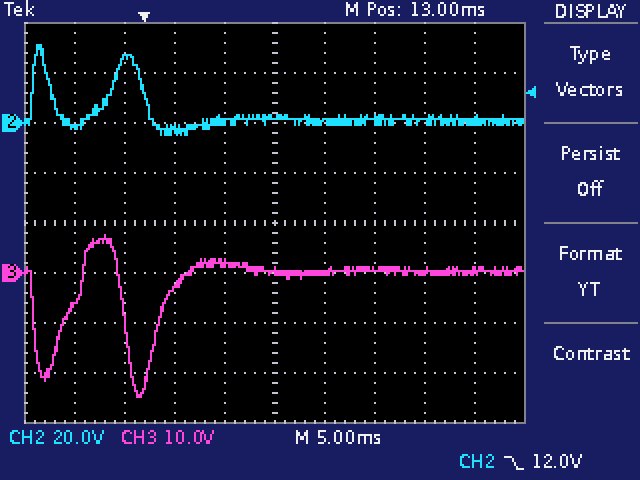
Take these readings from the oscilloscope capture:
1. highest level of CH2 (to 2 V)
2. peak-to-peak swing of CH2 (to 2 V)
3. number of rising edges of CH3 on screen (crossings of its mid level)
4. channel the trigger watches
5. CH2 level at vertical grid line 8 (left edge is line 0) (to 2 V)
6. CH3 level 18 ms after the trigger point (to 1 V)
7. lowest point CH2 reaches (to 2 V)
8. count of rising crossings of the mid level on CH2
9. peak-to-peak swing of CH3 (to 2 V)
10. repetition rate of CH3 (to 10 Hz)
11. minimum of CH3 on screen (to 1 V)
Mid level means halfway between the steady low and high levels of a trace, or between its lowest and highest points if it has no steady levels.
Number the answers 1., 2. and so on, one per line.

1. 32 V
2. 36 V
3. 2
4. CH2
5. 0 V
6. 0 V
7. -4 V
8. 2
9. 32 V
10. 110 Hz
11. -25 V
